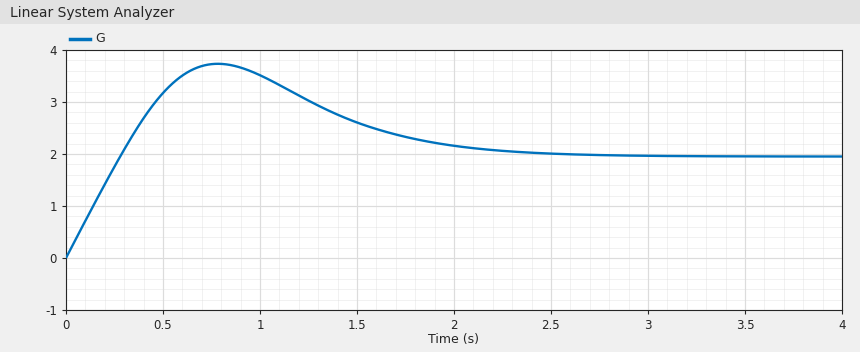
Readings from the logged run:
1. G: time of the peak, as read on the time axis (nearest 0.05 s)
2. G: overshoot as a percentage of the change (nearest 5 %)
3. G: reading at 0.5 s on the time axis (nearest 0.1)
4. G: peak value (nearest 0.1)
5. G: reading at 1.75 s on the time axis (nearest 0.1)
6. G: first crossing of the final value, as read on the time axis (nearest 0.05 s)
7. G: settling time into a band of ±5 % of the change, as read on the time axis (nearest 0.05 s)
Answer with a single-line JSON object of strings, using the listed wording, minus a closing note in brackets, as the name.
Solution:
{"G: time of the peak, as read on the time axis": "0.80 s", "G: overshoot as a percentage of the change": "90 %", "G: reading at 0.5 s on the time axis": "3.2", "G: peak value": "3.7", "G: reading at 1.75 s on the time axis": "2.3", "G: first crossing of the final value, as read on the time axis": "0.30 s", "G: settling time into a band of ±5 % of the change, as read on the time axis": "2.30 s"}
